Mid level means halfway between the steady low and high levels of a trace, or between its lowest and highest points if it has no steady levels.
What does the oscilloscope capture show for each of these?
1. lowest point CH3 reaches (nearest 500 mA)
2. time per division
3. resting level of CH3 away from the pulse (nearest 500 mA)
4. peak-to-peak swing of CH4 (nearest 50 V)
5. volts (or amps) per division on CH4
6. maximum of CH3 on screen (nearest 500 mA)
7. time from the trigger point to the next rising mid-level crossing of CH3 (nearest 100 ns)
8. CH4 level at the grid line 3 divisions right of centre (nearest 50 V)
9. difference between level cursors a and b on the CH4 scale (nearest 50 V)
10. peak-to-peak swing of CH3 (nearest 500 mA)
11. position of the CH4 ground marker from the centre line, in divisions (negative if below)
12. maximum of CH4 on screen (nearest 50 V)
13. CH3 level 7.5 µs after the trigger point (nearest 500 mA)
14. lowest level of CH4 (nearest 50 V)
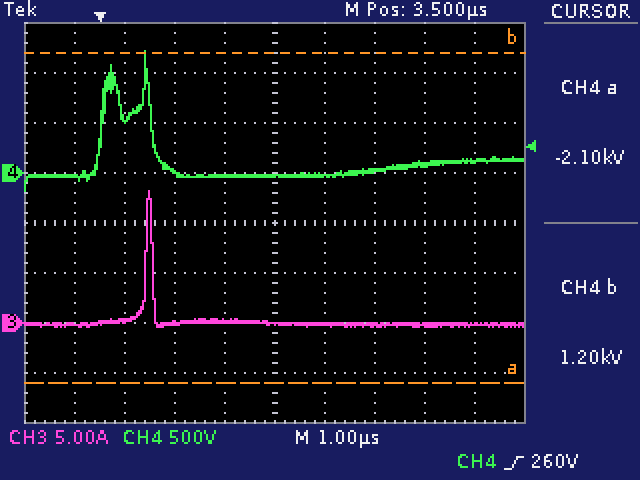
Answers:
-500 mA
1 µs
0.0 A
1.40 kV
500 V
13.0 A
900 ns
100 V
3.30 kV
13.5 A
+1.0 div
1.20 kV
0.0 A
-200 V
